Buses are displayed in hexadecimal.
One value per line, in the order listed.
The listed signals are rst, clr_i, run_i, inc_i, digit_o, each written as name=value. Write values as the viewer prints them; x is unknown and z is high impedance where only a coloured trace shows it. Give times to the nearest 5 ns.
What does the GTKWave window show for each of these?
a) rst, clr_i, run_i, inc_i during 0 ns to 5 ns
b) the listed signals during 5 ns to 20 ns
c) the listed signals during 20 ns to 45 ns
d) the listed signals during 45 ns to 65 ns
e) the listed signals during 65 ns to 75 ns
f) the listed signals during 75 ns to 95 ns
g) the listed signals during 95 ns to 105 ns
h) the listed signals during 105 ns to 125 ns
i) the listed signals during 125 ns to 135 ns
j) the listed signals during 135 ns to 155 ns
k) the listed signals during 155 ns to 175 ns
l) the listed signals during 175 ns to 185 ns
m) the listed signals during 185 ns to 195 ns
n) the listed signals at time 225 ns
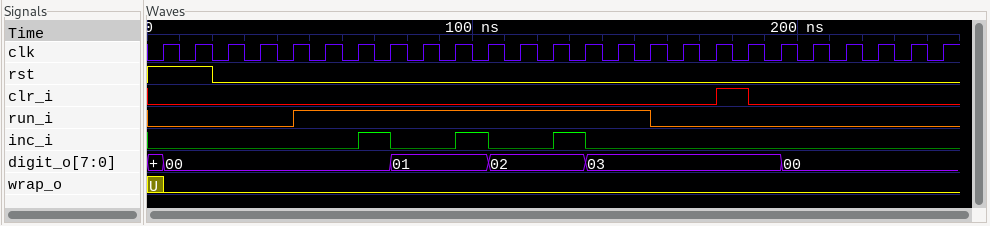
rst=1, clr_i=0, run_i=0, inc_i=0
rst=1, clr_i=0, run_i=0, inc_i=0, digit_o=00
rst=0, clr_i=0, run_i=0, inc_i=0, digit_o=00
rst=0, clr_i=0, run_i=1, inc_i=0, digit_o=00
rst=0, clr_i=0, run_i=1, inc_i=1, digit_o=00
rst=0, clr_i=0, run_i=1, inc_i=0, digit_o=01
rst=0, clr_i=0, run_i=1, inc_i=1, digit_o=01
rst=0, clr_i=0, run_i=1, inc_i=0, digit_o=02
rst=0, clr_i=0, run_i=1, inc_i=1, digit_o=02
rst=0, clr_i=0, run_i=1, inc_i=0, digit_o=03
rst=0, clr_i=0, run_i=0, inc_i=0, digit_o=03
rst=0, clr_i=1, run_i=0, inc_i=0, digit_o=03
rst=0, clr_i=0, run_i=0, inc_i=0, digit_o=03
rst=0, clr_i=0, run_i=0, inc_i=0, digit_o=00
